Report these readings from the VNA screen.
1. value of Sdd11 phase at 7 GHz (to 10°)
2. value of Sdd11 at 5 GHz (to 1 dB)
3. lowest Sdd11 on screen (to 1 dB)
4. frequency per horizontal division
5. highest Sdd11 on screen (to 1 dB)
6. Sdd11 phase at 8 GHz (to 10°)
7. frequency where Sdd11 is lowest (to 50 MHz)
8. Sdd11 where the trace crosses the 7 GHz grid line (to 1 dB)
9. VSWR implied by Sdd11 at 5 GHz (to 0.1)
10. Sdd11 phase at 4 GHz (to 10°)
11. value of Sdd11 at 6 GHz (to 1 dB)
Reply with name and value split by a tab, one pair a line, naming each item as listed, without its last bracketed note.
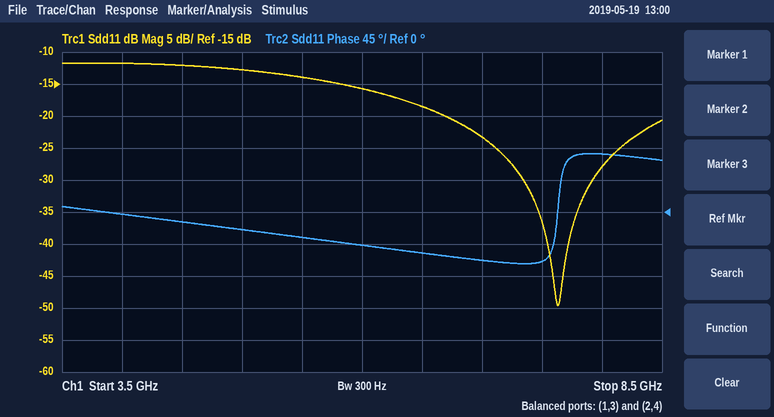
value of Sdd11 phase at 7 GHz	-70°
value of Sdd11 at 5 GHz	-13 dB
lowest Sdd11 on screen	-50 dB
frequency per horizontal division	500 MHz
highest Sdd11 on screen	-12 dB
Sdd11 phase at 8 GHz	80°
frequency where Sdd11 is lowest	7.65 GHz
Sdd11 where the trace crosses the 7 GHz grid line	-23 dB
VSWR implied by Sdd11 at 5 GHz	1.6
Sdd11 phase at 4 GHz	0°
value of Sdd11 at 6 GHz	-16 dB
